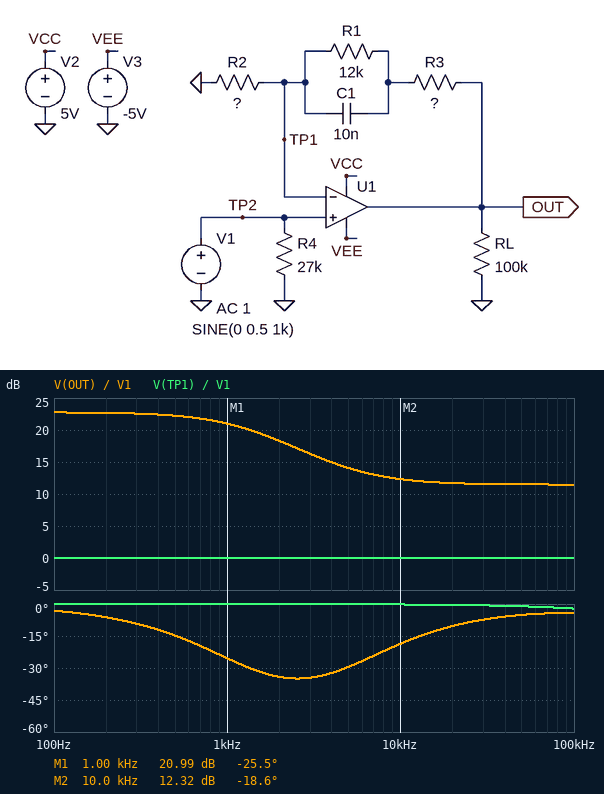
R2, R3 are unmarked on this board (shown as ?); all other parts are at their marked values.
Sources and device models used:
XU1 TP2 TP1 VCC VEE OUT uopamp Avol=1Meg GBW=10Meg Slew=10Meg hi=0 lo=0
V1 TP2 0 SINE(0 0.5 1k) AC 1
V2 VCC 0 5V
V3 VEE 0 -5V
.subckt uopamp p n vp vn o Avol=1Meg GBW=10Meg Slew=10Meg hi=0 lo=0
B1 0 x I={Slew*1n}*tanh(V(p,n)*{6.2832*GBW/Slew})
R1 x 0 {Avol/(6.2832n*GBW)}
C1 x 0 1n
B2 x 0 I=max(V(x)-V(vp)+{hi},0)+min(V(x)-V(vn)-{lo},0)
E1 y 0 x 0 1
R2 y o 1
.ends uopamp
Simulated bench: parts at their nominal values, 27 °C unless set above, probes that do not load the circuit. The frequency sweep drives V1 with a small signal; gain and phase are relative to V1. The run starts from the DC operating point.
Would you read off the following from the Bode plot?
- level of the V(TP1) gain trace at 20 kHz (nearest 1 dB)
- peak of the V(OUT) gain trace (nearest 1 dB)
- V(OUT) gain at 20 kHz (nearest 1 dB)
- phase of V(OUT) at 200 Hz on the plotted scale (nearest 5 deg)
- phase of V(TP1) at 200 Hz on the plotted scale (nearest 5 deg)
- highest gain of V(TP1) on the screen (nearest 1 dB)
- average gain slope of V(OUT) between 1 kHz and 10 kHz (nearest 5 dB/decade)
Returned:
0 dB
23 dB
12 dB
-5 deg
0 deg
0 dB
-10 dB/decade
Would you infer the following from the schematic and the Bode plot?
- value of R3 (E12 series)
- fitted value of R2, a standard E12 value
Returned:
3.3 kΩ
1.2 kΩ
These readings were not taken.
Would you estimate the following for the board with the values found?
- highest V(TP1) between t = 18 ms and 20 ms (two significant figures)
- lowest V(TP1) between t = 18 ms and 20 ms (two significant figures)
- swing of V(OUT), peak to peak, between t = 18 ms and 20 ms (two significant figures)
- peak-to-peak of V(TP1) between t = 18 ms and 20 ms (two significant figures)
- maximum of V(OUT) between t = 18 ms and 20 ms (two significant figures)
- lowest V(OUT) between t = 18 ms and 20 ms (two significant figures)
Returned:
500 mV
-500 mV
10 V
1.0 V
5.0 V
-5.0 V
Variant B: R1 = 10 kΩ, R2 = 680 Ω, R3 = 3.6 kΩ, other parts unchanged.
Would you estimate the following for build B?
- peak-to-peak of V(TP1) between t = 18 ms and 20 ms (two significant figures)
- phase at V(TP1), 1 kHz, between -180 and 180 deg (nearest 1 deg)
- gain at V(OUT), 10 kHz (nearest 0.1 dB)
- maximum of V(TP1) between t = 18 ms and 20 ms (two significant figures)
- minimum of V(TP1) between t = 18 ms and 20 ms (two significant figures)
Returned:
800 mV
0 deg
16.9 dB
400 mV
-400 mV
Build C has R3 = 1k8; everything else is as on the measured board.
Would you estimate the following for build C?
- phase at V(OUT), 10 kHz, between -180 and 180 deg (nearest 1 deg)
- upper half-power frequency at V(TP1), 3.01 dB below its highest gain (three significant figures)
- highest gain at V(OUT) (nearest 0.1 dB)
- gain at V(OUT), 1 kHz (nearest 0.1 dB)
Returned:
-26 deg
3.99 MHz
21.9 dB
20.1 dB
